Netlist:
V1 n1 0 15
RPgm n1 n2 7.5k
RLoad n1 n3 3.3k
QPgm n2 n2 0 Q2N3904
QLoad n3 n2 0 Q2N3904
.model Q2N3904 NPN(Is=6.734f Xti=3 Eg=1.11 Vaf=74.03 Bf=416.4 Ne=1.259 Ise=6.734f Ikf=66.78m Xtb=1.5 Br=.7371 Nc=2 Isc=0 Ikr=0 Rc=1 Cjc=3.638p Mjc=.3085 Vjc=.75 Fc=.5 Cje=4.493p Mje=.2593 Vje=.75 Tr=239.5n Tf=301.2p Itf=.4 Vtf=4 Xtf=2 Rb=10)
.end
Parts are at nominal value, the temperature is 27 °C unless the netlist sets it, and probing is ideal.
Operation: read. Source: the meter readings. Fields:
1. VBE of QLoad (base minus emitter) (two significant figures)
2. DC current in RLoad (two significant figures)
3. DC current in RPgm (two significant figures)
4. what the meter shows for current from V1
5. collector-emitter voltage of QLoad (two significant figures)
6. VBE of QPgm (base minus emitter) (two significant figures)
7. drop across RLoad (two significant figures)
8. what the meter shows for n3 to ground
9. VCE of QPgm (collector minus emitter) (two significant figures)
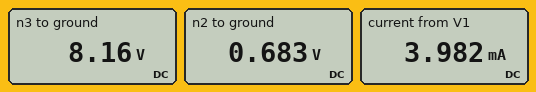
680 mV
2.1 mA
1.9 mA
3.982 mA
8.2 V
680 mV
6.8 V
8.16 V
680 mV
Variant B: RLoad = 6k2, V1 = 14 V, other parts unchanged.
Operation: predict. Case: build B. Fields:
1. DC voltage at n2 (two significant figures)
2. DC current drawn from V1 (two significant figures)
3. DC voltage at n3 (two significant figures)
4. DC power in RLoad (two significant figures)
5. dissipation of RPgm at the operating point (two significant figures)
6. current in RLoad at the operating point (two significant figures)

680 mV
3.6 mA
2.8 V
20 mW
24 mW
1.8 mA
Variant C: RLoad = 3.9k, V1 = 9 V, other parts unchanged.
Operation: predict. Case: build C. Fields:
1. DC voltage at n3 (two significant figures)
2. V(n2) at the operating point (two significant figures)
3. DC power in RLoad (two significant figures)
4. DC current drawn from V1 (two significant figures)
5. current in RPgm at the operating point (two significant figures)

4.5 V
670 mV
5.2 mW
2.3 mA
1.1 mA
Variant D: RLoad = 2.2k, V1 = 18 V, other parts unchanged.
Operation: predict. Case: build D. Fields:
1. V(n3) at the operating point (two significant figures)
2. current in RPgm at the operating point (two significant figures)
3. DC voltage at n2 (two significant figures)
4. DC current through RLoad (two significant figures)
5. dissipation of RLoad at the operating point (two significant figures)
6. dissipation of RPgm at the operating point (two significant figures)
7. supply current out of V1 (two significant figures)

12 V
2.3 mA
690 mV
2.6 mA
15 mW
40 mW
4.9 mA
